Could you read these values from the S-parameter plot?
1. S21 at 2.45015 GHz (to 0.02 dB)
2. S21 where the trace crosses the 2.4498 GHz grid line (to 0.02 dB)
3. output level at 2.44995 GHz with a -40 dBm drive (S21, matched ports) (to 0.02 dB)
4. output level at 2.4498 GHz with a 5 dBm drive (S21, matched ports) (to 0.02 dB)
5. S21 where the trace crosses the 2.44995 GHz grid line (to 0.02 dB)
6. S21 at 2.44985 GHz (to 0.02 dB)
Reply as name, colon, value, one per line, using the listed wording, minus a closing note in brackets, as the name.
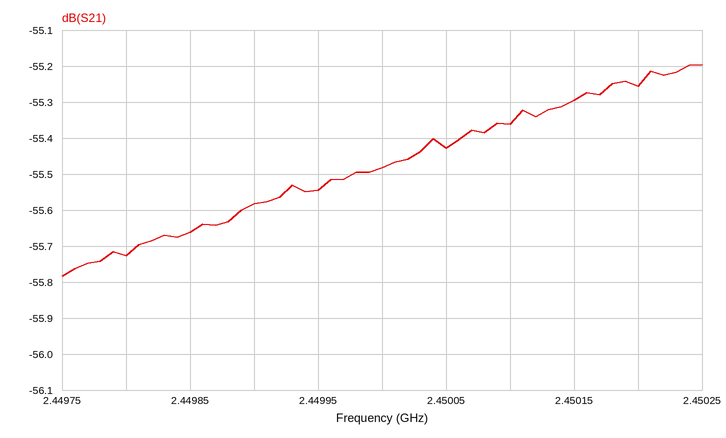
S21 at 2.45015 GHz: -55.30 dB
S21 where the trace crosses the 2.4498 GHz grid line: -55.72 dB
output level at 2.44995 GHz with a -40 dBm drive (S21, matched ports): -95.54 dBm
output level at 2.4498 GHz with a 5 dBm drive (S21, matched ports): -50.72 dBm
S21 where the trace crosses the 2.44995 GHz grid line: -55.54 dB
S21 at 2.44985 GHz: -55.66 dB
